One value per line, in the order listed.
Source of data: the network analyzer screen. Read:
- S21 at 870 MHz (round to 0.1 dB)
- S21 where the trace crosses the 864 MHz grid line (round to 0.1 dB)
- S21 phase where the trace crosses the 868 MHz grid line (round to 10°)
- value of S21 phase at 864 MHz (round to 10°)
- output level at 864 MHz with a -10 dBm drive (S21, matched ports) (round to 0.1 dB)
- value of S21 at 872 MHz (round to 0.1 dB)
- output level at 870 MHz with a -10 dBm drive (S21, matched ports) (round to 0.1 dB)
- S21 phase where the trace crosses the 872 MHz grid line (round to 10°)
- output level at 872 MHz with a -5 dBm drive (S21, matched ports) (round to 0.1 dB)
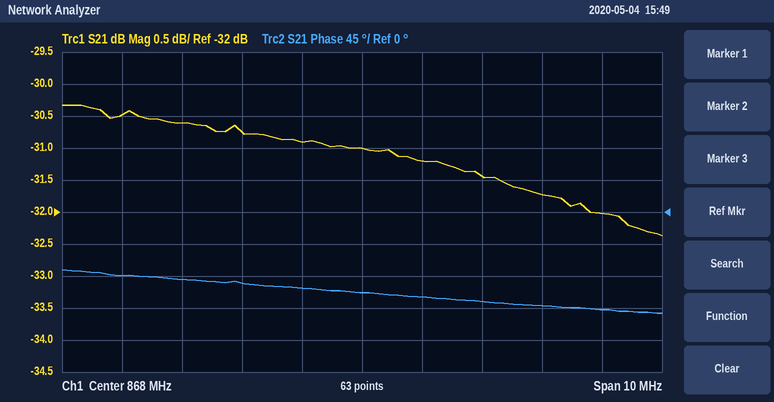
-31.4 dB
-30.5 dB
-110°
-90°
-40.5 dBm
-32.0 dB
-41.4 dBm
-140°
-37.0 dBm
